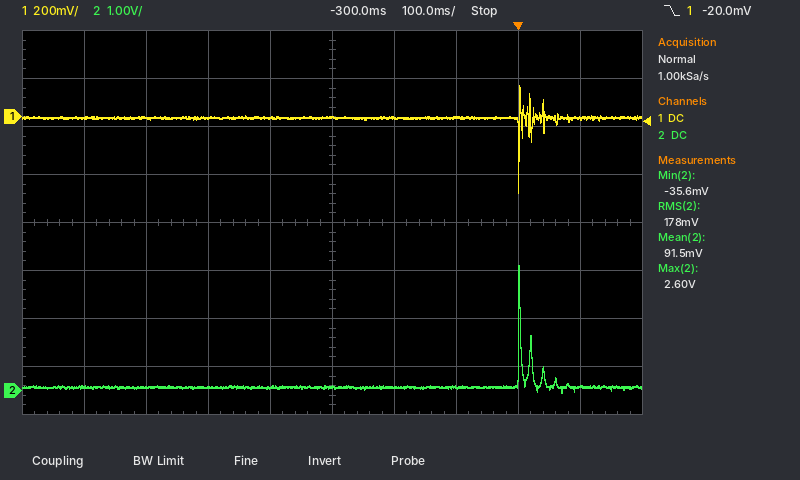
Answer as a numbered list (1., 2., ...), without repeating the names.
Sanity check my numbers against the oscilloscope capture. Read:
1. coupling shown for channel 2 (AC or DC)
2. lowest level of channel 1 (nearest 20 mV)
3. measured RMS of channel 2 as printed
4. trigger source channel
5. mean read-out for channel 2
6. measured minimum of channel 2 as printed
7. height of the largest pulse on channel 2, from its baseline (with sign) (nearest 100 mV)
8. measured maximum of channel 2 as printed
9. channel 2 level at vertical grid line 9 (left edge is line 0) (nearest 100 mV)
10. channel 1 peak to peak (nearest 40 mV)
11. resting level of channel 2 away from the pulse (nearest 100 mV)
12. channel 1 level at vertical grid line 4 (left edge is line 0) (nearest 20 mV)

1. DC
2. -320 mV
3. 178 mV
4. channel 1
5. 91.5 mV
6. -35.6 mV
7. +2.5 V
8. 2.60 V
9. 100 mV
10. 440 mV
11. 100 mV
12. 0 mV
